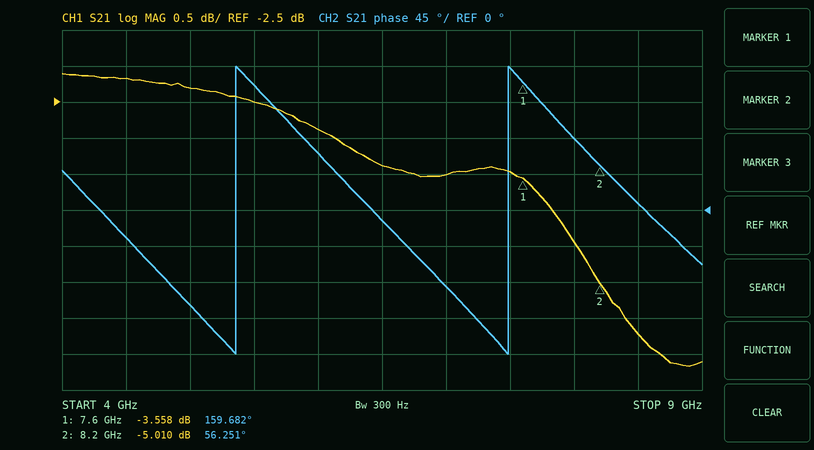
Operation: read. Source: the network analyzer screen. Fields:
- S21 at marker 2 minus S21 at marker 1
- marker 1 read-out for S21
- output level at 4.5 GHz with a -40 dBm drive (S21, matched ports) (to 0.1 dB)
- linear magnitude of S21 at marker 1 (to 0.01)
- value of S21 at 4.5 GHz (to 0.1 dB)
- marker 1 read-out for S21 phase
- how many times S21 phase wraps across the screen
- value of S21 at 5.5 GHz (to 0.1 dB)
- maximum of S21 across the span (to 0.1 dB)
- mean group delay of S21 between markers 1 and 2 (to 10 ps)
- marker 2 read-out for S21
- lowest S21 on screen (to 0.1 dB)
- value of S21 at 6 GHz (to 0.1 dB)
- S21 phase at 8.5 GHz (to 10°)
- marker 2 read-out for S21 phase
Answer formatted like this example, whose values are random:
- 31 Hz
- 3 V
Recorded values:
- -1.452 dB
- -3.558 dB
- -42.2 dBm
- 0.66
- -2.2 dB
- 159.682°
- 2
- -2.5 dB
- -2.1 dB
- 480 ps
- -5.010 dB
- -6.2 dB
- -2.9 dB
- 10°
- 56.251°
